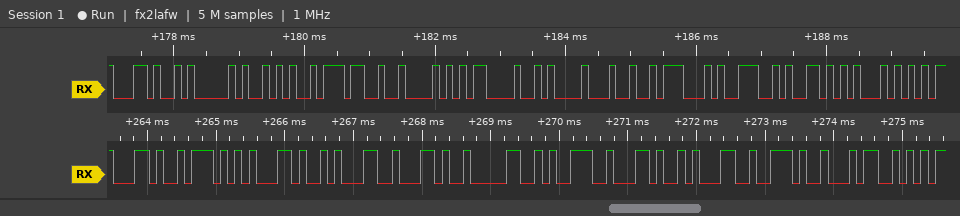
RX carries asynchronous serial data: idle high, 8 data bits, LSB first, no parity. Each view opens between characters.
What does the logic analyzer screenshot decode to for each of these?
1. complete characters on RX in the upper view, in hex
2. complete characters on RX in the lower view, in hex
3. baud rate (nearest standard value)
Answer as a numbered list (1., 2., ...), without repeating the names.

1. 2C, 41, 2A, 37, 42, 0D, 0A, 24, 47, 4E, 56, 54
2. 2C, 57, 2C, 31, 2C, 30, 39, 2C, 31, 2E, 34
3. 9600 baud
